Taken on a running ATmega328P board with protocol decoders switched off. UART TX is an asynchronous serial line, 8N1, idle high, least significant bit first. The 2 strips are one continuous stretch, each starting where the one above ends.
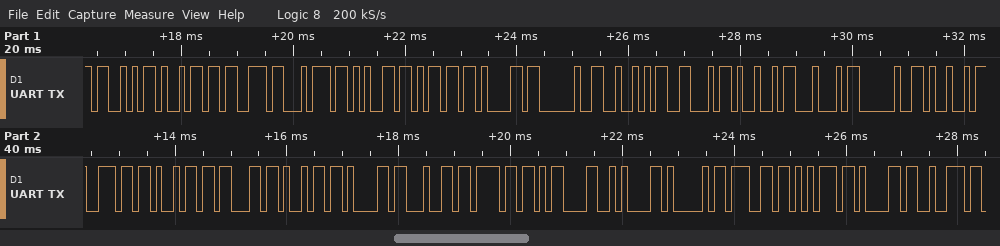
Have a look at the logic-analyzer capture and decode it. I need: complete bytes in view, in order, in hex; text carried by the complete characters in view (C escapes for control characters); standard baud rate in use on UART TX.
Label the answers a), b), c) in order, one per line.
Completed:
a) 53 69 73 74 65 6D 61 20 52 46 49 44 20 49 6E 69 63 69 61 64 6F 0D 0A 41 67 75 61 72
b) "Sistema RFID Iniciado\r\nAguar"
c) 9600 baud
